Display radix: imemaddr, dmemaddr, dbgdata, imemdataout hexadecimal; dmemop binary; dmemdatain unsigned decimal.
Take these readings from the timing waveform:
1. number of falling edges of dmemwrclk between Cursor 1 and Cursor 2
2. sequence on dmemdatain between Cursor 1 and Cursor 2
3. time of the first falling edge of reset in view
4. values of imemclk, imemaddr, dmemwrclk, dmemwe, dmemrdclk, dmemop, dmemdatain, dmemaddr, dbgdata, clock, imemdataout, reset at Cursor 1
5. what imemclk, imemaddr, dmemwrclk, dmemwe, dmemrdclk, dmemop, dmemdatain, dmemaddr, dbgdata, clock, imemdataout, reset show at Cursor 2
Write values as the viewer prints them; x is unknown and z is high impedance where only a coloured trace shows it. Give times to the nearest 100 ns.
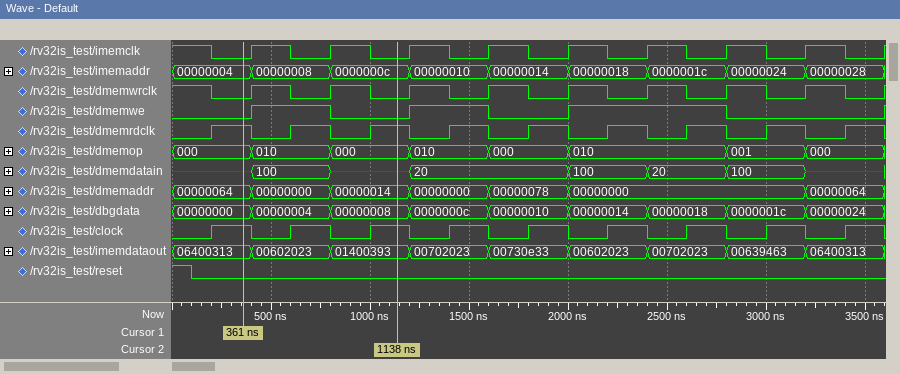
2
x, 100, x
100 ns
imemclk=0, imemaddr=00000004, dmemwrclk=0, dmemwe=0, dmemrdclk=1, dmemop=000, dmemdatain=x, dmemaddr=00000064, dbgdata=00000000, clock=1, imemdataout=06400313, reset=0
imemclk=0, imemaddr=0000000c, dmemwrclk=0, dmemwe=0, dmemrdclk=1, dmemop=000, dmemdatain=x, dmemaddr=00000014, dbgdata=00000008, clock=1, imemdataout=01400393, reset=0
